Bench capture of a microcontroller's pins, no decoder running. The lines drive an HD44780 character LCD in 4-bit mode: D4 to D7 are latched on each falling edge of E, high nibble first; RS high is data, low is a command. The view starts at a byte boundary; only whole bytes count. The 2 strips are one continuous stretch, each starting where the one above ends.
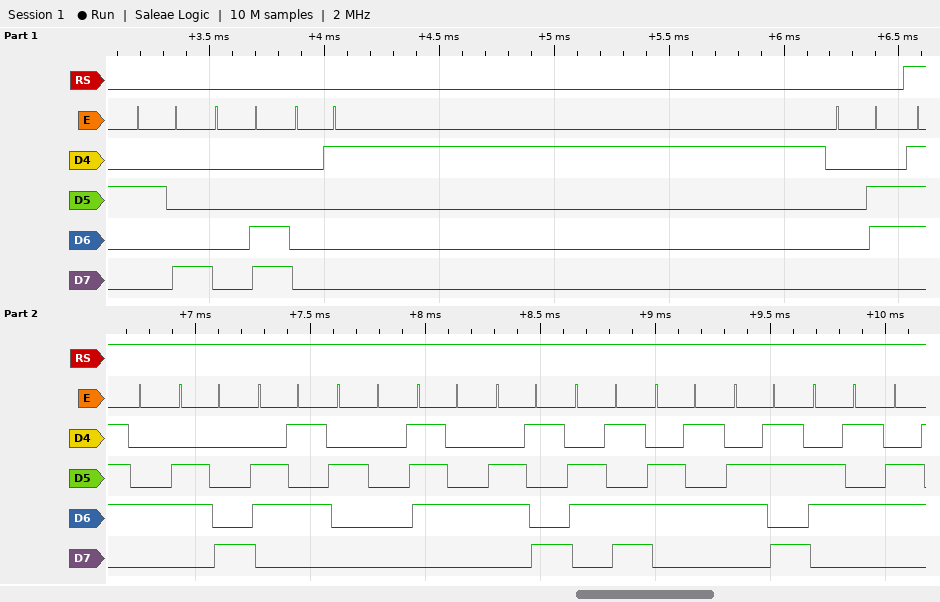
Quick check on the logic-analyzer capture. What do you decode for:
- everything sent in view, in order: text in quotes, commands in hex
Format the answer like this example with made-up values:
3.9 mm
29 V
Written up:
0x28 0x0C 0x01 0x06 "the timeke"
